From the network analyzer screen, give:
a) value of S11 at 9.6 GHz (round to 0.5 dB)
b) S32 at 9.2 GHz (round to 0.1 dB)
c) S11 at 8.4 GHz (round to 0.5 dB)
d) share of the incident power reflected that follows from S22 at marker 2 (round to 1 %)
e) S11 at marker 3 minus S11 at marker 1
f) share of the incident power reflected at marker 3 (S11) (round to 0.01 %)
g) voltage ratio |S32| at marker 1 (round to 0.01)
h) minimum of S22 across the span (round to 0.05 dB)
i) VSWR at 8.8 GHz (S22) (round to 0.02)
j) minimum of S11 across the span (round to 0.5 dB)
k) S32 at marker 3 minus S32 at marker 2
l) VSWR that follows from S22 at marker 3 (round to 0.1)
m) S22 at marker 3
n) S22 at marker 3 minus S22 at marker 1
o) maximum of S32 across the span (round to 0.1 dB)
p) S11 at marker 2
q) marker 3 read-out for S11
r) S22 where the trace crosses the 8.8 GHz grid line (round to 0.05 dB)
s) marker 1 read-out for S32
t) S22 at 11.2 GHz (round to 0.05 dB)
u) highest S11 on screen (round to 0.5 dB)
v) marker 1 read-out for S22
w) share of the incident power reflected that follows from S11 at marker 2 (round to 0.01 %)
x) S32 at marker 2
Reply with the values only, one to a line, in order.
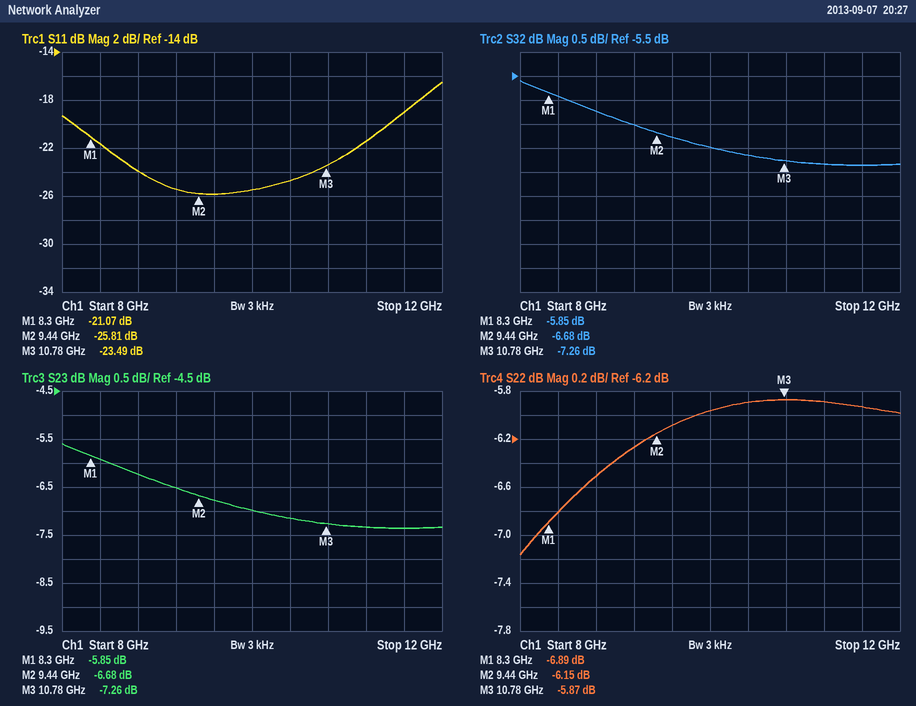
-26.0 dB
-6.5 dB
-21.5 dB
24 %
-2.42 dB
0.45 %
0.51
-7.15 dB
2.80
-26.0 dB
-0.58 dB
3.1
-5.87 dB
1.02 dB
-5.6 dB
-25.81 dB
-23.49 dB
-6.50 dB
-5.85 dB
-5.90 dB
-16.5 dB
-6.89 dB
0.26 %
-6.68 dB
